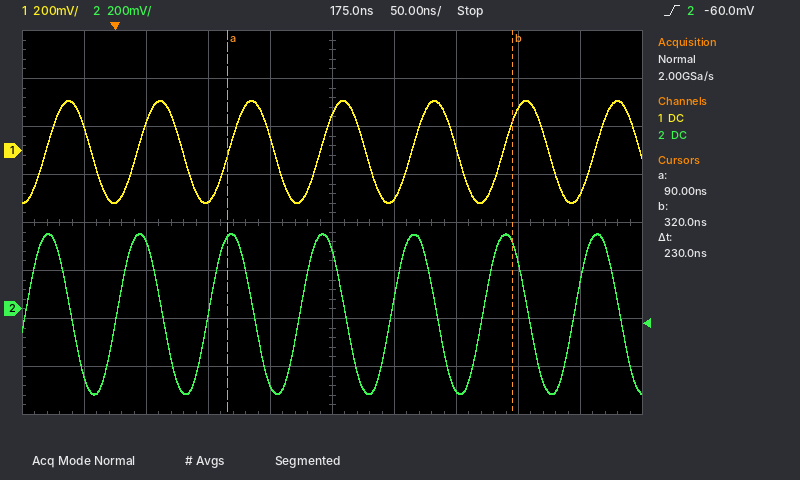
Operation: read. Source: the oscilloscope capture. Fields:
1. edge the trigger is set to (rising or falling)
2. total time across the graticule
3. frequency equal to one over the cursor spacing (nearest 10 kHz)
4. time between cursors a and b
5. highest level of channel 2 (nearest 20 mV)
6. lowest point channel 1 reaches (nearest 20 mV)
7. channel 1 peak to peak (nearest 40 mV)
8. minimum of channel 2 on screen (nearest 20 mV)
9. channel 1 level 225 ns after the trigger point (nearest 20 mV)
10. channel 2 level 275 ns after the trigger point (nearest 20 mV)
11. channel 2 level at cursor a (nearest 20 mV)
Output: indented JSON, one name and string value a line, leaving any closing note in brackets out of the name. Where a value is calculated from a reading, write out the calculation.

{
  "edge the trigger is set to": "rising",
  "total time across the graticule": "500 ns",
  "frequency equal to one over the cursor spacing": "1 / 230 ns ≈ 4.35 MHz",
  "time between cursors a and b": "230 ns",
  "highest level of channel 2": "320 mV",
  "lowest point channel 1 reaches": "-220 mV",
  "channel 1 peak to peak": "440 mV",
  "minimum of channel 2 on screen": "-360 mV",
  "channel 1 level 225 ns after the trigger point": "-200 mV",
  "channel 2 level 275 ns after the trigger point": "-340 mV",
  "channel 2 level at cursor a": "300 mV"
}
